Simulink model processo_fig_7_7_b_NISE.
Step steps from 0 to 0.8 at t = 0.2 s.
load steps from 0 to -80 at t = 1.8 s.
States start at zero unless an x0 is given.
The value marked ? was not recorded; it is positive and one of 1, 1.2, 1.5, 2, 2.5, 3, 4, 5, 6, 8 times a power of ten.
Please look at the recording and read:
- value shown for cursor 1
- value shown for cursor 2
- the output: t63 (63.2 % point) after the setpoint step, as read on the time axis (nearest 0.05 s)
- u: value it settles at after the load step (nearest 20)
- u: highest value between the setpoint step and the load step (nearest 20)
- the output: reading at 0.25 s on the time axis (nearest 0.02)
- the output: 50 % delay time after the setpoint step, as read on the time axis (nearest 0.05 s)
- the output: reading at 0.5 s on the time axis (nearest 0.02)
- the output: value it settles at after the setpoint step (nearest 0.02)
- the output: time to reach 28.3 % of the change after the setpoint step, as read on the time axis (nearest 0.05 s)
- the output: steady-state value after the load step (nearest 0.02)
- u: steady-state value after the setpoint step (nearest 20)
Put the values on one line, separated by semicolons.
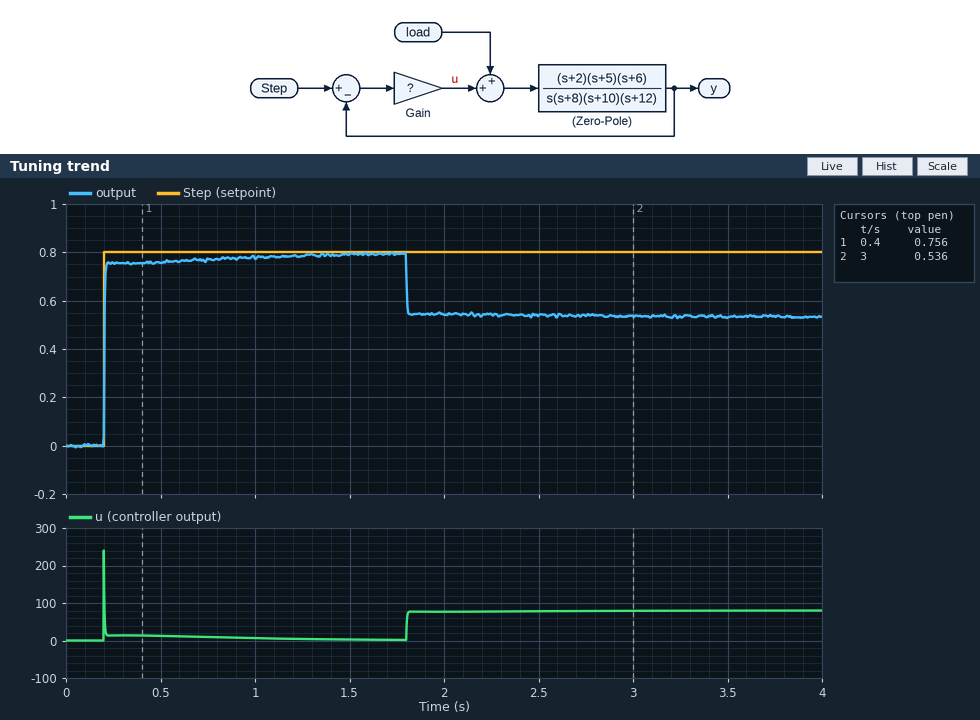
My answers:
0.756; 0.536; 0.20 s; 80; 240; 0.76; 0.20 s; 0.76; 0.80; 0.20 s; 0.54; 0
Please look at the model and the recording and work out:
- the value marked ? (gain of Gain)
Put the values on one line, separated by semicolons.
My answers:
300
